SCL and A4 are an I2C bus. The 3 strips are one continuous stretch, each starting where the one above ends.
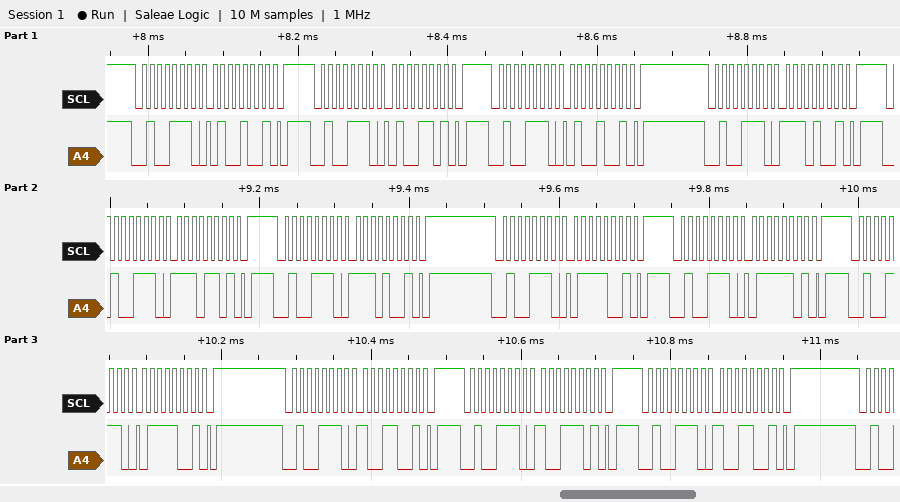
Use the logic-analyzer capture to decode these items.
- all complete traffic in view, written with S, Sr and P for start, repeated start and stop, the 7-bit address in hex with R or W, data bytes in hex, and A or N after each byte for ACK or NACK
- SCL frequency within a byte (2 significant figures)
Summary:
S 27W A 49 A P S 27W A 4D A P S 27W A 49 A P S 27W A E9 A P S 27W A ED A P S 27W A E9 A P S 27W A 79 A P S 27W A 7D A P S 27W A 79 A P S 27W A 99 A P S 27W A 9D A P S 27W A 99 A P
100 kHz
